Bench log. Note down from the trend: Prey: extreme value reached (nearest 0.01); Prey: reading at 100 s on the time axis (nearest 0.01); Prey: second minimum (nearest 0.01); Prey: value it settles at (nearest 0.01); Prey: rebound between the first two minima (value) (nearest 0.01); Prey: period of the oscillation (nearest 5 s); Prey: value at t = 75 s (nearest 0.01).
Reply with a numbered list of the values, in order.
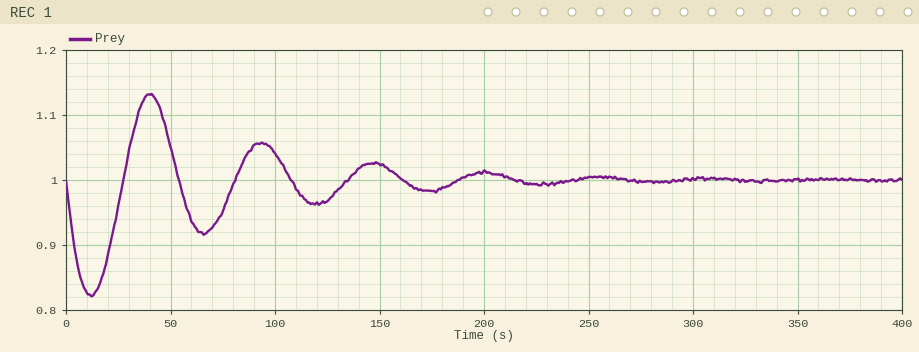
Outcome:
1. 0.82
2. 1.04
3. 0.92
4. 1.00
5. 1.13
6. 55 s
7. 0.95
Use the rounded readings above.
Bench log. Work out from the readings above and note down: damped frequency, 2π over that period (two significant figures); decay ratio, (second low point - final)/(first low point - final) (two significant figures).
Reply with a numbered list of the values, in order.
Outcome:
1. 0.11 rad/s
2. 0.44
